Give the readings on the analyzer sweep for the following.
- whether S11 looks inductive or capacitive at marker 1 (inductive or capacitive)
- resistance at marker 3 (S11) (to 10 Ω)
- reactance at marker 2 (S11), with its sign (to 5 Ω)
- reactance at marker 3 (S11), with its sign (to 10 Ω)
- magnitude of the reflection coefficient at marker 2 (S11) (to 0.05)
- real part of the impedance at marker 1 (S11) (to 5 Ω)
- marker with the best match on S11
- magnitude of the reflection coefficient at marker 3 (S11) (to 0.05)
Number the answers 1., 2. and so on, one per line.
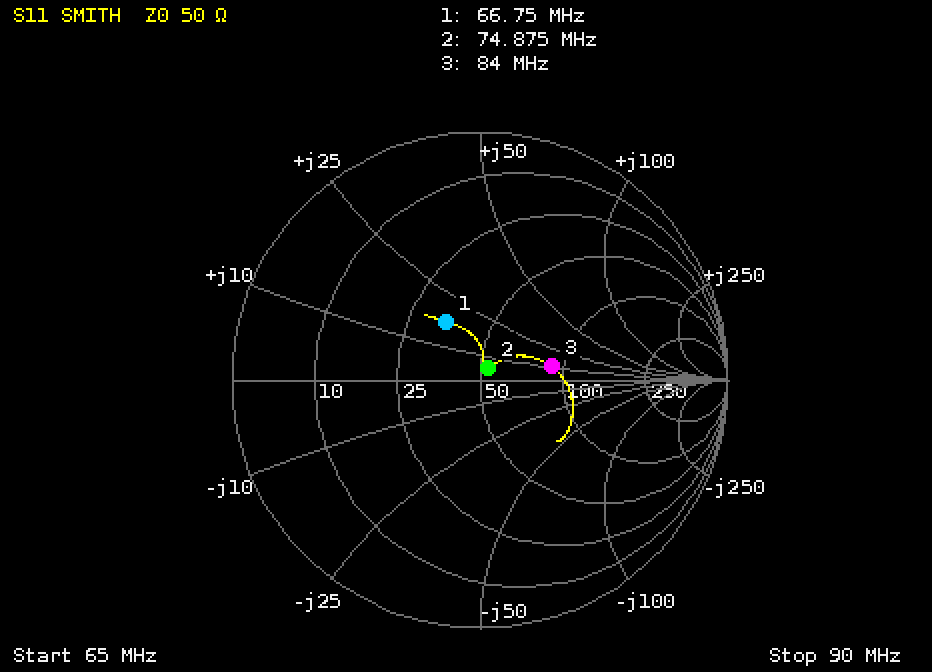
1. inductive
2. 90 Ω
3. +5 Ω
4. +10 Ω
5. 0.05
6. 35 Ω
7. marker 2
8. 0.30
